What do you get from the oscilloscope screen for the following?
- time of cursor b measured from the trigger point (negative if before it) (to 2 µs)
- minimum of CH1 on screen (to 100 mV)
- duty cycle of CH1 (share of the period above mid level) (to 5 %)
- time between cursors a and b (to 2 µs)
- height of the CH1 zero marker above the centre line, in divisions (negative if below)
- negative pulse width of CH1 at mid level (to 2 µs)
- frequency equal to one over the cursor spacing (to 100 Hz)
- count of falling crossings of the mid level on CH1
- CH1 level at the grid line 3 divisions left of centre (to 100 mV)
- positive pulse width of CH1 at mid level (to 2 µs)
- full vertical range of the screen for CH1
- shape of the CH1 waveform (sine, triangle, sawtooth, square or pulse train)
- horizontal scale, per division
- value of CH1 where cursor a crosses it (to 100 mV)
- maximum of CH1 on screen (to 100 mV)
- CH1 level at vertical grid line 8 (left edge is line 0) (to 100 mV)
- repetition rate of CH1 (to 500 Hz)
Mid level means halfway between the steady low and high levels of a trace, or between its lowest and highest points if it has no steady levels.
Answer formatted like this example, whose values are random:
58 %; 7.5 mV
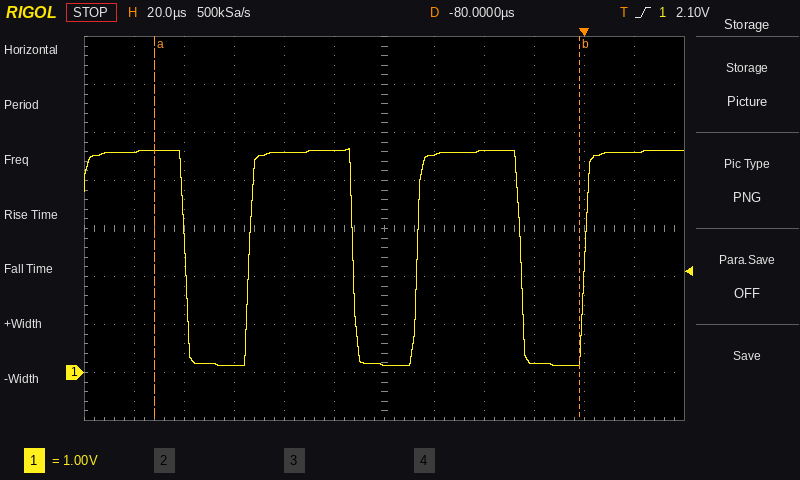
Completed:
-2 µs; 100 mV; 60 %; 170 µs; -3.0 div; 26 µs; 5.9 kHz; 3; 100 mV; 42 µs; 8 V; pulse train; 20 µs; 4.6 V; 4.7 V; 4.6 V; 15.0 kHz
